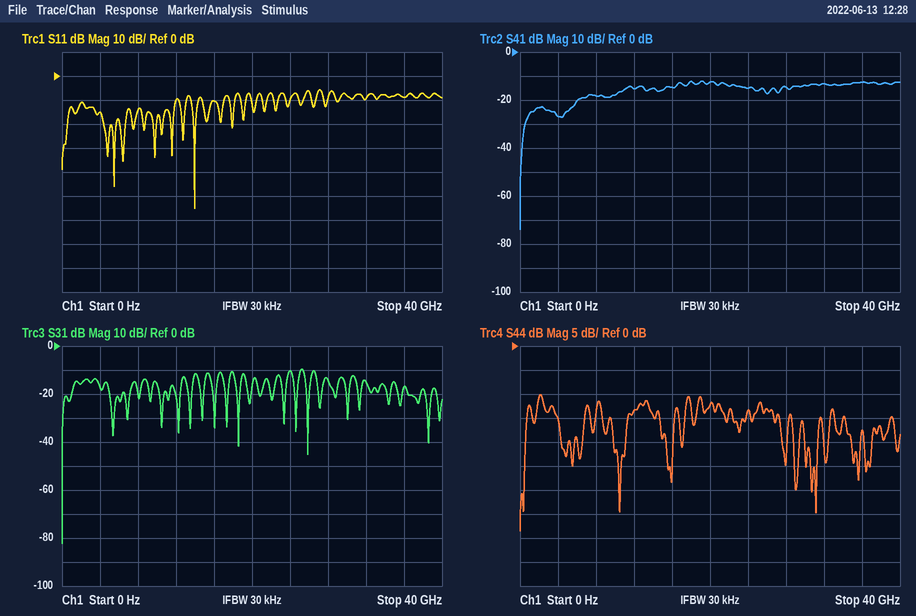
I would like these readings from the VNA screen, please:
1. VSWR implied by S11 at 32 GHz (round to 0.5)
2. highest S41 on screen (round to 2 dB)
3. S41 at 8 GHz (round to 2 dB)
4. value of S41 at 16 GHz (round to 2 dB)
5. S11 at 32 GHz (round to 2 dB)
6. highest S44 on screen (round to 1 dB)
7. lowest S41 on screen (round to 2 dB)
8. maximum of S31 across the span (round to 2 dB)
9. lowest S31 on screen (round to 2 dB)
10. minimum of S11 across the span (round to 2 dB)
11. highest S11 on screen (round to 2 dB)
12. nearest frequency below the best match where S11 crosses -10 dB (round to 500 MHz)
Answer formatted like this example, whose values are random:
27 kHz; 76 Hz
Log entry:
2.0; -12 dB; -18 dB; -14 dB; -10 dB; -10 dB; -74 dB; -10 dB; -82 dB; -56 dB; -6 dB; 13.5 GHz
